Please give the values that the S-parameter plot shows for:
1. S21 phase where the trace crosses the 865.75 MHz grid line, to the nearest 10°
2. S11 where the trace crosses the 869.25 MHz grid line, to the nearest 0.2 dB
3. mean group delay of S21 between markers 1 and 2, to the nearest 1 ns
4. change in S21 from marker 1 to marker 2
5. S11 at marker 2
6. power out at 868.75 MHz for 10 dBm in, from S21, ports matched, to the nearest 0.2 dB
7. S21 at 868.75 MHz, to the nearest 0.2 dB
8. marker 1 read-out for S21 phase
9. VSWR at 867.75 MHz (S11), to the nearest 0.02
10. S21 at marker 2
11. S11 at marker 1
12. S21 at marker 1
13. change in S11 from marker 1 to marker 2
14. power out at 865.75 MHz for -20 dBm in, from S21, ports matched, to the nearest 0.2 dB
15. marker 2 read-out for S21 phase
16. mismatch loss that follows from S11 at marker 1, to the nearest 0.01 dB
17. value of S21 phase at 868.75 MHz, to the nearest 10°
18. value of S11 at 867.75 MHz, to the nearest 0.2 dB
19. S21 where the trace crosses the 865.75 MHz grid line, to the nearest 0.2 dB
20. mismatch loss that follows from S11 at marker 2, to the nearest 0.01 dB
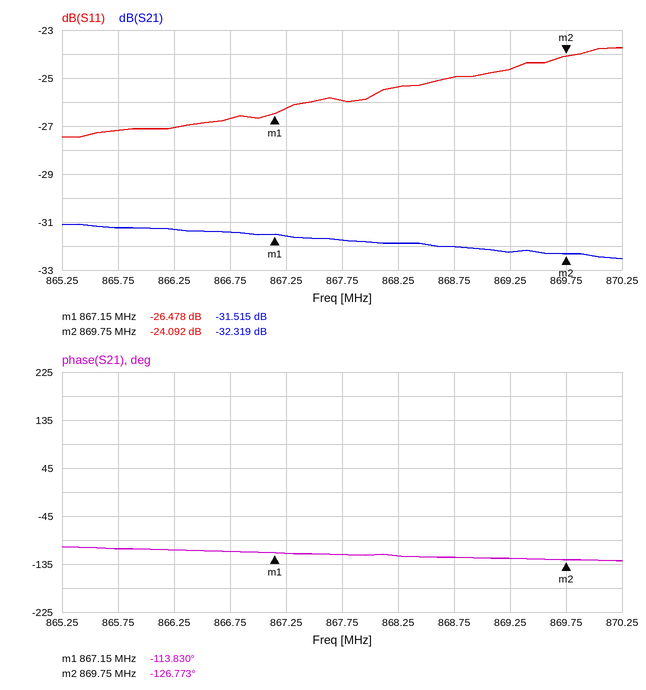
-110°
-24.6 dB
14 ns
-0.804 dB
-24.092 dB
-22.0 dBm
-32.0 dB
-113.830°
1.10
-32.319 dB
-26.478 dB
-31.515 dB
2.386 dB
-51.2 dBm
-126.773°
0.01 dB
-120°
-26.0 dB
-31.2 dB
0.02 dB
